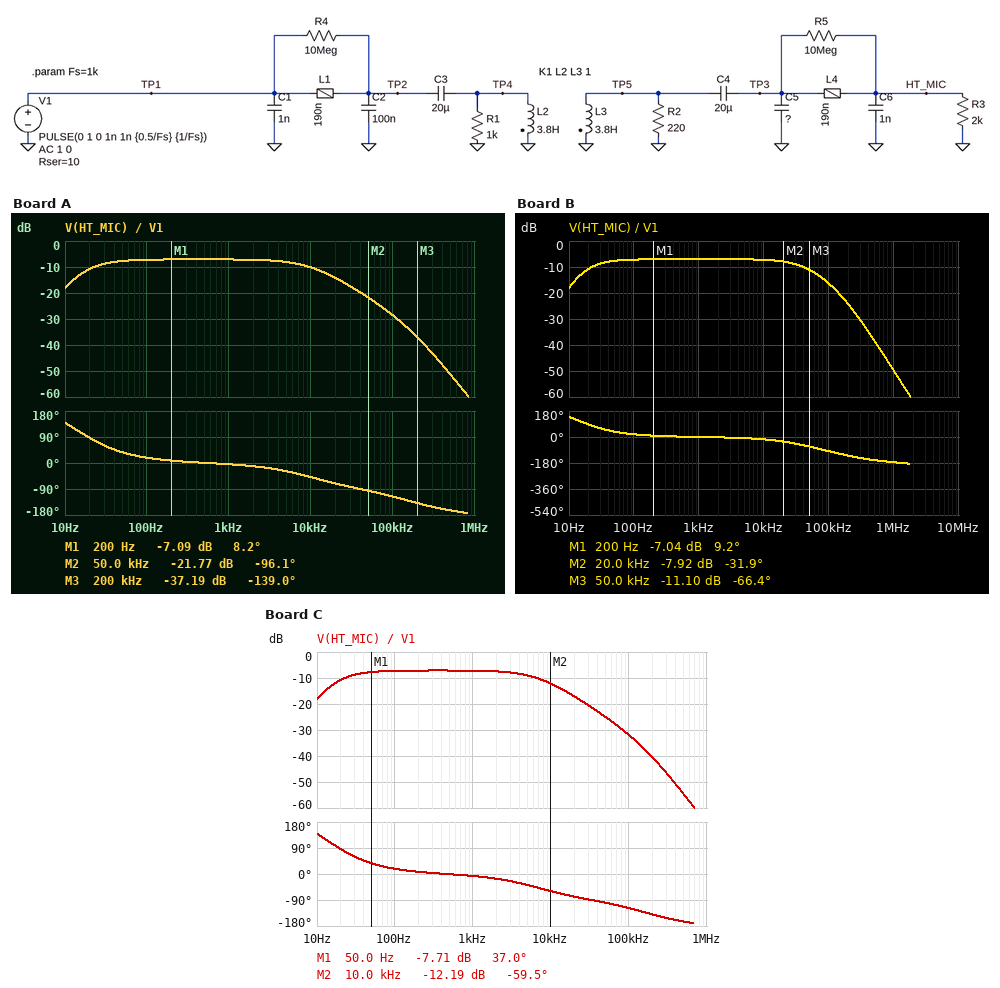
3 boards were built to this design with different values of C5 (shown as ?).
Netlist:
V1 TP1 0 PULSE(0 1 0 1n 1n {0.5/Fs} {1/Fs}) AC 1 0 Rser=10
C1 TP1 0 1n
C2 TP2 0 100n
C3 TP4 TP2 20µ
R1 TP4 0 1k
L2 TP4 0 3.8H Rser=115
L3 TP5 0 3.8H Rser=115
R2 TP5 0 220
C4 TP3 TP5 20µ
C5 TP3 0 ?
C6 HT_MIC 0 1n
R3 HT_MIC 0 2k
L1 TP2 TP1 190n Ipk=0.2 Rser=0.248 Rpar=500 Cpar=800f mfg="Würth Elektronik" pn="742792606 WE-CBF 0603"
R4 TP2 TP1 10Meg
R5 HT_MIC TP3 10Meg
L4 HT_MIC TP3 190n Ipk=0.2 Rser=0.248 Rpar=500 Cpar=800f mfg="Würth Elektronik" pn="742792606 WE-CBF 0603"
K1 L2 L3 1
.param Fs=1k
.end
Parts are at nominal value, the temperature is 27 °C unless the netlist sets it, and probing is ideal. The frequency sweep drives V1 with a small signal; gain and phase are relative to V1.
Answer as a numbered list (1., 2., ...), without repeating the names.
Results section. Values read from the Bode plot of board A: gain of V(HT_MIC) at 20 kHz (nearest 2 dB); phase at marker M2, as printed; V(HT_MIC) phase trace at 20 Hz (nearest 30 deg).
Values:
1. -14 dB
2. -96.1 deg
3. 90 deg
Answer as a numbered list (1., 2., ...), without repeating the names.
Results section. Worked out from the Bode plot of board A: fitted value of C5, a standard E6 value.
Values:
1. 150 nF
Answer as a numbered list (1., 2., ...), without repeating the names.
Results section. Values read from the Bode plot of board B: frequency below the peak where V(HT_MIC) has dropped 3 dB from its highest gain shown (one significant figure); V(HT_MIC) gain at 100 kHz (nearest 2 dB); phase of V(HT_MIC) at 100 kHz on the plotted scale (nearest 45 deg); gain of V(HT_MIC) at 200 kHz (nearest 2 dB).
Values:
1. 20 Hz
2. -16 dB
3. -90 deg
4. -24 dB
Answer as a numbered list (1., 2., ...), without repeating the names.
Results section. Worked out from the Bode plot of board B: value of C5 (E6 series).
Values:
1. 33 nF
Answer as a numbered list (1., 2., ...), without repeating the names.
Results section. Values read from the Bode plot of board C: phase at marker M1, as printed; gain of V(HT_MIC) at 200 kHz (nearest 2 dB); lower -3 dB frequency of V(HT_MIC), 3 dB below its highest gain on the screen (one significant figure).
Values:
1. 37.0 deg
2. -40 dB
3. 20 Hz
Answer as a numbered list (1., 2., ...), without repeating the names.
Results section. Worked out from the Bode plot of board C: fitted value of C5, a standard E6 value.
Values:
1. 220 nF
